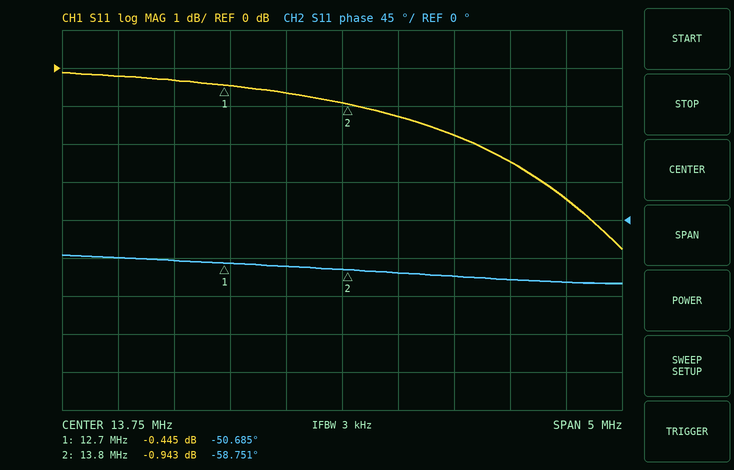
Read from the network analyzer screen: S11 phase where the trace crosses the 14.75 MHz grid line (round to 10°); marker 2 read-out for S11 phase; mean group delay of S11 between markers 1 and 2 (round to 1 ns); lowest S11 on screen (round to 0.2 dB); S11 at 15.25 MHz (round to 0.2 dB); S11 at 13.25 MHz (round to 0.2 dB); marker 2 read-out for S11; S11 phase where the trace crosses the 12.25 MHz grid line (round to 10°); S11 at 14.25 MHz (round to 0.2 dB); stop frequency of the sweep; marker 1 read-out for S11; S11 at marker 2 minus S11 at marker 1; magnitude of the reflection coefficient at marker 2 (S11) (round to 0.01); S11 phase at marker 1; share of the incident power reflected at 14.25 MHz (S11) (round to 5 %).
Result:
-70°
-58.751°
20 ns
-4.8 dB
-2.4 dB
-0.6 dB
-0.943 dB
-50°
-1.2 dB
16.25 MHz
-0.445 dB
-0.498 dB
0.90
-50.685°
75 %
